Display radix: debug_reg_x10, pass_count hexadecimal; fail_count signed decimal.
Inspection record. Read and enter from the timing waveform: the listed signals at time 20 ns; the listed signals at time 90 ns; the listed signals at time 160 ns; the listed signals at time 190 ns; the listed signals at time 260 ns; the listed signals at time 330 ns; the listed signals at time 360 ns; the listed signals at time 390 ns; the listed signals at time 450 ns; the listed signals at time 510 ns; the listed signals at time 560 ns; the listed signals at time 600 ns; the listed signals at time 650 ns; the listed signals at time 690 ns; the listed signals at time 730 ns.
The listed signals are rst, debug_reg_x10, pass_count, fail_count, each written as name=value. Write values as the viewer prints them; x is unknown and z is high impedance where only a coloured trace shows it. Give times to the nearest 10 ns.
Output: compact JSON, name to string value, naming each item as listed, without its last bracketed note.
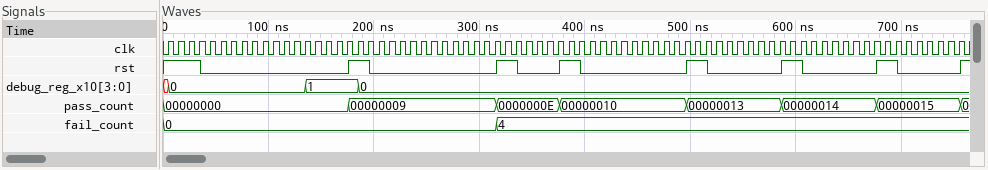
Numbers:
{"the listed signals at time 20 ns": "rst=1, debug_reg_x10=0, pass_count=00000000, fail_count=0", "the listed signals at time 90 ns": "rst=0, debug_reg_x10=0, pass_count=00000000, fail_count=0", "the listed signals at time 160 ns": "rst=0, debug_reg_x10=1, pass_count=00000000, fail_count=0", "the listed signals at time 190 ns": "rst=1, debug_reg_x10=0, pass_count=00000009, fail_count=0", "the listed signals at time 260 ns": "rst=0, debug_reg_x10=0, pass_count=00000009, fail_count=0", "the listed signals at time 330 ns": "rst=1, debug_reg_x10=0, pass_count=0000000E, fail_count=4", "the listed signals at time 360 ns": "rst=0, debug_reg_x10=0, pass_count=0000000E, fail_count=4", "the listed signals at time 390 ns": "rst=1, debug_reg_x10=0, pass_count=00000010, fail_count=4", "the listed signals at time 450 ns": "rst=0, debug_reg_x10=0, pass_count=00000010, fail_count=4", "the listed signals at time 510 ns": "rst=1, debug_reg_x10=0, pass_count=00000013, fail_count=4", "the listed signals at time 560 ns": "rst=0, debug_reg_x10=0, pass_count=00000013, fail_count=4", "the listed signals at time 600 ns": "rst=1, debug_reg_x10=0, pass_count=00000014, fail_count=4", "the listed signals at time 650 ns": "rst=0, debug_reg_x10=0, pass_count=00000014, fail_count=4", "the listed signals at time 690 ns": "rst=1, debug_reg_x10=0, pass_count=00000015, fail_count=4", "the listed signals at time 730 ns": "rst=0, debug_reg_x10=0, pass_count=00000015, fail_count=4"}
